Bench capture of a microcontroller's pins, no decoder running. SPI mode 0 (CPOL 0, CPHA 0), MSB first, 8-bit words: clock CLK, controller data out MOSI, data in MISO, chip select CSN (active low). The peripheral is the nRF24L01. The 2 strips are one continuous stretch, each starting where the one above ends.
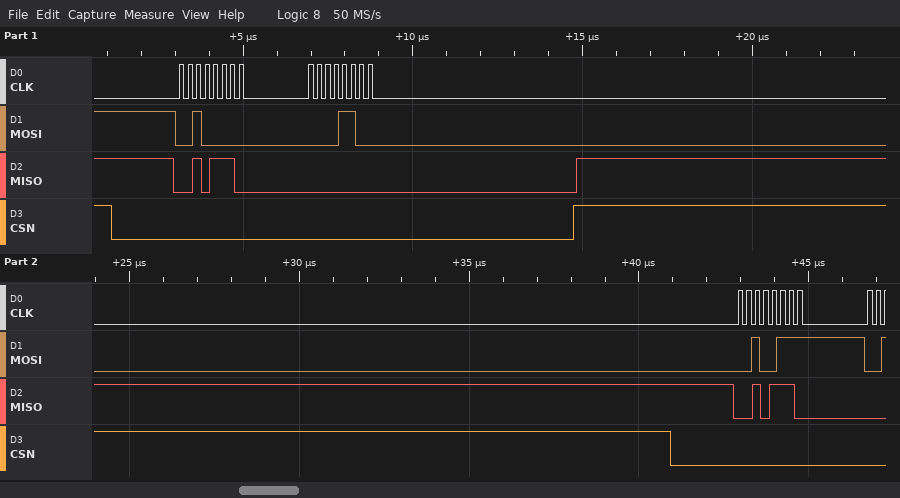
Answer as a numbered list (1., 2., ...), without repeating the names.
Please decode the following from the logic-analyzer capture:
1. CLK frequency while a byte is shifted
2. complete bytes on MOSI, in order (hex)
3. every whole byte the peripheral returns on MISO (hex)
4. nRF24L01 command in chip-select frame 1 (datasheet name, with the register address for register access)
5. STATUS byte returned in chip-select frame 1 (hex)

1. 4 MHz
2. 20 0C 27
3. 2E 00 2E
4. W_REGISTER 0x00
5. 0x2E
